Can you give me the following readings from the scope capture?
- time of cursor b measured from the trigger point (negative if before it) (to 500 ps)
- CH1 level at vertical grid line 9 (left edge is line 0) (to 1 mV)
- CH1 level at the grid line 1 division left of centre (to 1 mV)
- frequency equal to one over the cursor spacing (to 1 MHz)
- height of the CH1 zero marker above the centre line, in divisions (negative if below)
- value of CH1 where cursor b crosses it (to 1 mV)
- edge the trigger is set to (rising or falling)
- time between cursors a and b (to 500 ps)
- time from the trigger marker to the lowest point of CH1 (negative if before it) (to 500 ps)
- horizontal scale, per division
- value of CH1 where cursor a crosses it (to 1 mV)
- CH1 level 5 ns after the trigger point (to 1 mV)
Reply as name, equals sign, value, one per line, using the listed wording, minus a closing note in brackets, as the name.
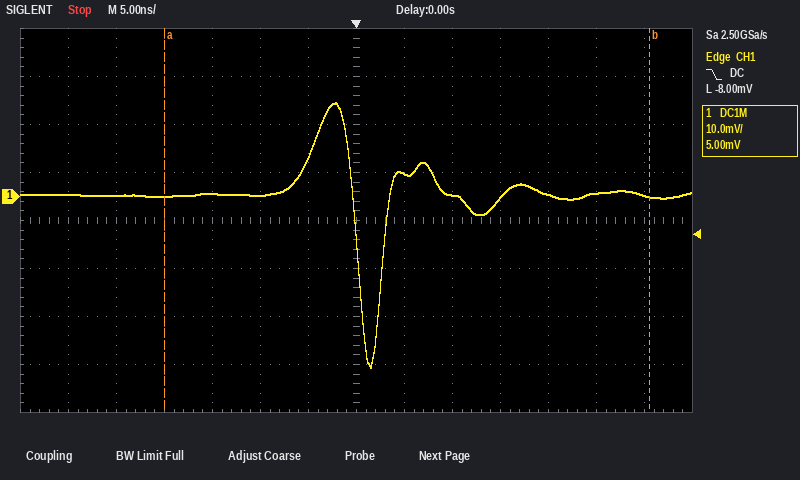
time of cursor b measured from the trigger point (negative if before it) = +30.5 ns
CH1 level at vertical grid line 9 (left edge is line 0) = 0 mV
CH1 level at the grid line 1 division left of centre = 8 mV
frequency equal to one over the cursor spacing = 20 MHz
height of the CH1 zero marker above the centre line, in divisions = +0.5 div
value of CH1 where cursor b crosses it = 0 mV
edge the trigger is set to = falling
time between cursors a and b = 50.5 ns
time from the trigger marker to the lowest point of CH1 (negative if before it) = +1.5 ns
horizontal scale, per division = 5 ns
value of CH1 where cursor a crosses it = 0 mV
CH1 level 5 ns after the trigger point = 5 mV
